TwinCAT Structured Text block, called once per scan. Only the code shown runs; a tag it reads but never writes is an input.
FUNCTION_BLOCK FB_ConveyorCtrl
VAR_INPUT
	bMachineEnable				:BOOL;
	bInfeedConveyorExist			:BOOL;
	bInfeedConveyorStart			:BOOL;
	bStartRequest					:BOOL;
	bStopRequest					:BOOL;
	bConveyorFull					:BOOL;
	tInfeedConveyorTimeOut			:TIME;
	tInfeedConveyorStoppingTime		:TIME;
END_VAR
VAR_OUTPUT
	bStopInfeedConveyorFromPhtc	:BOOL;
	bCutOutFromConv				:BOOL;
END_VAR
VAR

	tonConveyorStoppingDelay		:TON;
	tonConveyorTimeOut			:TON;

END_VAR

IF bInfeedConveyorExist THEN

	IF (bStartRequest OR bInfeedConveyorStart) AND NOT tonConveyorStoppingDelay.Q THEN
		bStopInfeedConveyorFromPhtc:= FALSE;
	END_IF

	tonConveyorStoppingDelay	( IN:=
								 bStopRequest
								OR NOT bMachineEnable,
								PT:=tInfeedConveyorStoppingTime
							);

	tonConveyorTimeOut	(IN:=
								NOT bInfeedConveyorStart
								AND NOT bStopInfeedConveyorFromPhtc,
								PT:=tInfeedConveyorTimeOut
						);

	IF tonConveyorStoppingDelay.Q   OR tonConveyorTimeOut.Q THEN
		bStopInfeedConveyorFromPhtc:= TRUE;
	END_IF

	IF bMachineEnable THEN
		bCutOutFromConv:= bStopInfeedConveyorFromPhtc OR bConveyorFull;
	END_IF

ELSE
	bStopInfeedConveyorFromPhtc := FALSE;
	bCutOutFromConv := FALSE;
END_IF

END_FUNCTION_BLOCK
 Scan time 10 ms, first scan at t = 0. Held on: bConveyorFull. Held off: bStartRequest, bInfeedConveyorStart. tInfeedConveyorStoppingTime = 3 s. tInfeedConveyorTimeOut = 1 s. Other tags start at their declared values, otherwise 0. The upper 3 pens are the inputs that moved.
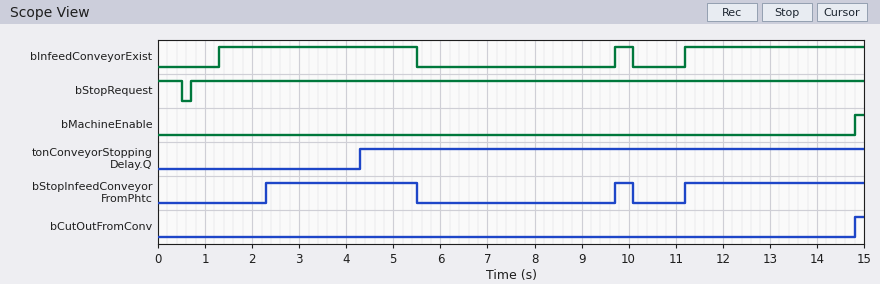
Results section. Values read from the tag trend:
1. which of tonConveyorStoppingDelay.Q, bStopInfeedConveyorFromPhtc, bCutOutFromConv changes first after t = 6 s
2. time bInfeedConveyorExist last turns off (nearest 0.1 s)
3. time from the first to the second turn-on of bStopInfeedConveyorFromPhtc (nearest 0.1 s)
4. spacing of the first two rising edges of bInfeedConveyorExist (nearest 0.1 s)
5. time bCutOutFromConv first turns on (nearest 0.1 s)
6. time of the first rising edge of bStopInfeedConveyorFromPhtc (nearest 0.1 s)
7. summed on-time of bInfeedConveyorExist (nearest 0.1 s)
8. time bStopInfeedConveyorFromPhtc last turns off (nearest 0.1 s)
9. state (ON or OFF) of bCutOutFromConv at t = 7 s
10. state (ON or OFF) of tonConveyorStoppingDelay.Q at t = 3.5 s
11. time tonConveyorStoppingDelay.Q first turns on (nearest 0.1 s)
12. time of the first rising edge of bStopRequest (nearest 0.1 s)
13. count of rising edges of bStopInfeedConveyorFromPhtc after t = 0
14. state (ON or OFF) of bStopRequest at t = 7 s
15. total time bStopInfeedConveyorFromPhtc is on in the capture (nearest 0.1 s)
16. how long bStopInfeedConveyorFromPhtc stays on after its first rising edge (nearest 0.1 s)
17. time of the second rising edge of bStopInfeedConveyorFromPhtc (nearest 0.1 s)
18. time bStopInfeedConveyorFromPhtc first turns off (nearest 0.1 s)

bStopInfeedConveyorFromPhtc
10.1 s
7.4 s
8.4 s
14.8 s
2.3 s
8.4 s
10.1 s
OFF
OFF
4.3 s
0.7 s
3
ON
7.4 s
3.2 s
9.7 s
5.5 s
